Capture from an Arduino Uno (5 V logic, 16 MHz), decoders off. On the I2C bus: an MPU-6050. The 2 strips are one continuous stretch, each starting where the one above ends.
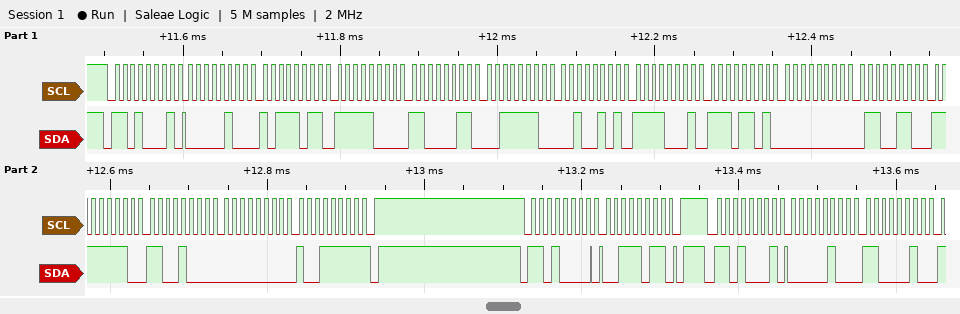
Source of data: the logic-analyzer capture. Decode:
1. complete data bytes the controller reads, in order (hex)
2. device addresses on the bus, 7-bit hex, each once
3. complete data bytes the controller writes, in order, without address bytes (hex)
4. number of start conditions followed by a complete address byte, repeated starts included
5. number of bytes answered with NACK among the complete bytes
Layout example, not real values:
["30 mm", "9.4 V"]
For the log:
["04 BB F8 C3 3E 25 F1 ED 00 66 FE C8 00 9F 04 C2", "0x68", "3B", "3", "1"]
